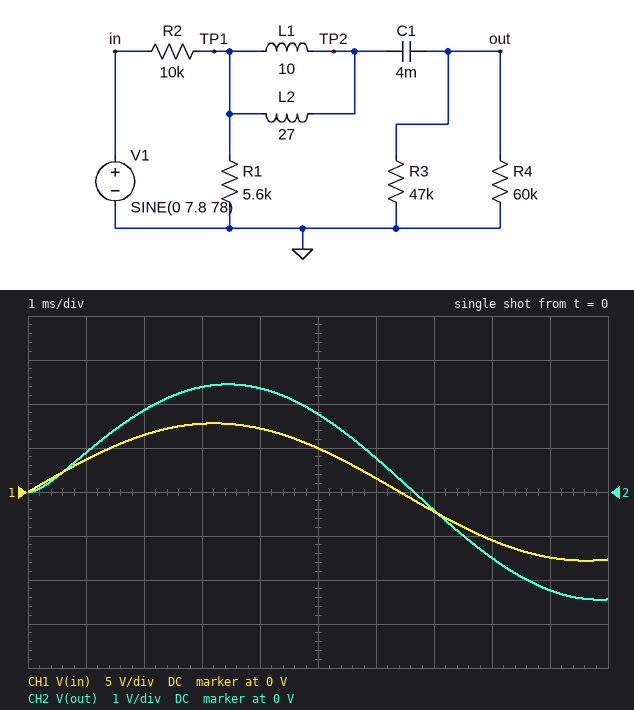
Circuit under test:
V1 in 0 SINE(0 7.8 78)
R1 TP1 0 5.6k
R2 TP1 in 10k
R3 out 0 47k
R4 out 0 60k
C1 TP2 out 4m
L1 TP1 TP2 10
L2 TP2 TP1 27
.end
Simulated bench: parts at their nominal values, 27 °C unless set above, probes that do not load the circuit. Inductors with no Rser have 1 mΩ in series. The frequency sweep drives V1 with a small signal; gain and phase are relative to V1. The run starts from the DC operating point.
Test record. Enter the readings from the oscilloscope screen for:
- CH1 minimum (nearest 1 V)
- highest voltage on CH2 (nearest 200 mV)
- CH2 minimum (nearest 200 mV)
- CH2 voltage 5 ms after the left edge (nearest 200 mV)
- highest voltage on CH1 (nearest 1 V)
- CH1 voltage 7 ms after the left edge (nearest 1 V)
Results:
-8 V
2.4 V
-2.4 V
1.8 V
8 V
-2 V
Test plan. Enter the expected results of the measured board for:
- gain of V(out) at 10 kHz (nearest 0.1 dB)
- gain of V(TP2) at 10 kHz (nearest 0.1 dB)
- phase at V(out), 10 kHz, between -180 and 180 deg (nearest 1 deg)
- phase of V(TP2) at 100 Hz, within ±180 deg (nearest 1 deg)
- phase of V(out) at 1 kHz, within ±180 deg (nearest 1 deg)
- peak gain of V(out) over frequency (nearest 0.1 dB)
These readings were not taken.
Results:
-33.7 dB
-33.7 dB
-86 deg
-9 deg
-57 deg
-10.0 dB
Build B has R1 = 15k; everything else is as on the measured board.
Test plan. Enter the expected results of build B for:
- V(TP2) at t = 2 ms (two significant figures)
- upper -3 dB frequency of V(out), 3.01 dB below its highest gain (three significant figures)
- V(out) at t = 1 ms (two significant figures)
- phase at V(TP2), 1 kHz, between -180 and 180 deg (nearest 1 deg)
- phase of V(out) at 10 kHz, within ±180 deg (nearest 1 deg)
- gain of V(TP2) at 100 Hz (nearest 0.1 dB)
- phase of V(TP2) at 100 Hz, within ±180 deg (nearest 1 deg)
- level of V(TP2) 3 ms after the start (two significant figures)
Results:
2.9 V
706 Hz
1.4 V
-55 deg
-86 deg
-6.3 dB
-8 deg
3.7 V
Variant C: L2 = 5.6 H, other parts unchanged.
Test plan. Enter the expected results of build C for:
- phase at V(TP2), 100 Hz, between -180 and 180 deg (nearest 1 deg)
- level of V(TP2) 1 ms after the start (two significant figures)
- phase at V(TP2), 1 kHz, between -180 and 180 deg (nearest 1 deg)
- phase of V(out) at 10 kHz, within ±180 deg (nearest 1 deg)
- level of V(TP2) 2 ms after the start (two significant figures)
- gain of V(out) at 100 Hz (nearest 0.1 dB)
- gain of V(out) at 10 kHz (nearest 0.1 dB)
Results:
-4 deg
1.0 V
-37 deg
-82 deg
2.0 V
-10.0 dB
-27.6 dB
